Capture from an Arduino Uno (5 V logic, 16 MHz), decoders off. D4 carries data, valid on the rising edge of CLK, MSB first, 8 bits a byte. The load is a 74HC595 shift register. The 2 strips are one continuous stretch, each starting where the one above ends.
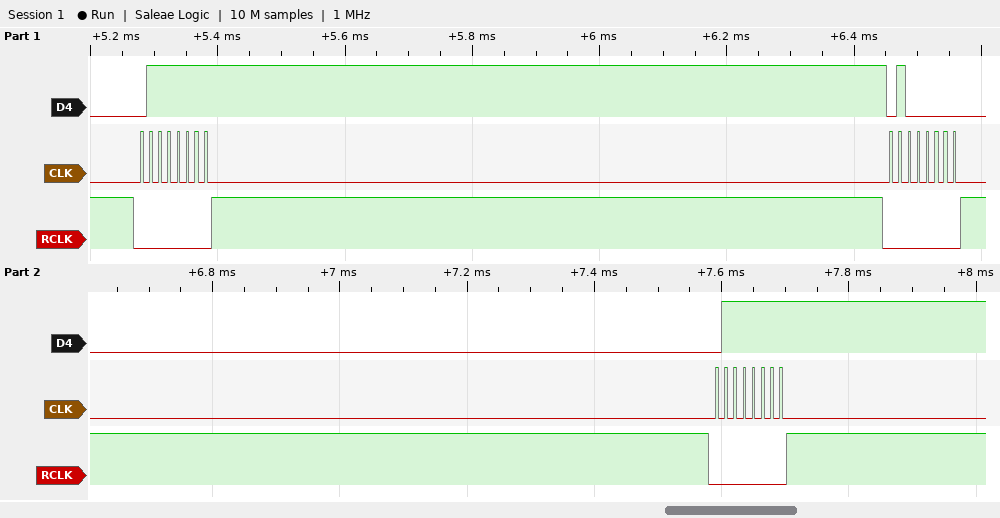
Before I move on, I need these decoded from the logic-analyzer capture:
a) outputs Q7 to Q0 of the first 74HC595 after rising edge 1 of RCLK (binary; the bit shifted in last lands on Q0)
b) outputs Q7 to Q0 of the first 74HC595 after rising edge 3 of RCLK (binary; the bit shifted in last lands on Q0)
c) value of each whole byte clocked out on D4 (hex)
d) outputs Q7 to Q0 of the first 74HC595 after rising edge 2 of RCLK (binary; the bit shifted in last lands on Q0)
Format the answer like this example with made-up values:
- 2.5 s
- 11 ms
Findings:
- 01111111
- 01111111
- 7F 40 7F
- 01000000
